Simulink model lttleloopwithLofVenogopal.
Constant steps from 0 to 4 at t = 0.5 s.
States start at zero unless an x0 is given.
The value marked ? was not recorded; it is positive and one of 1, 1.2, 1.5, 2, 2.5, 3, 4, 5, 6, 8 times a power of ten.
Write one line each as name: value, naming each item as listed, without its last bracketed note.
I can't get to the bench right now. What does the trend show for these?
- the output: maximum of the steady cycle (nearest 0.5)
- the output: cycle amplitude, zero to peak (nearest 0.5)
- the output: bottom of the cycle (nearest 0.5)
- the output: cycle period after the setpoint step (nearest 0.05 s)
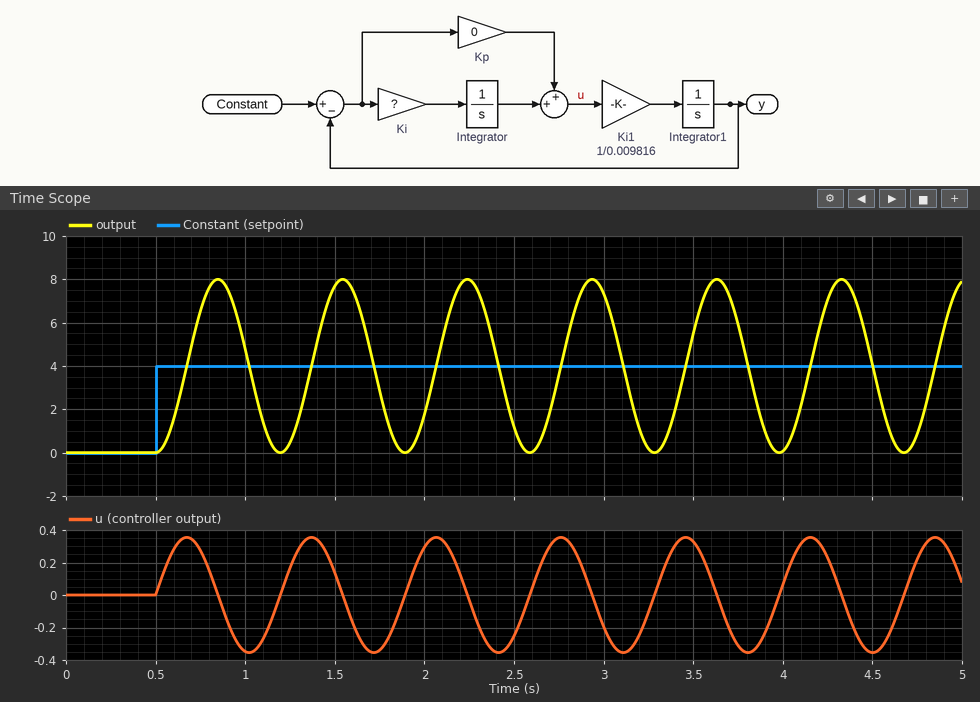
the output: maximum of the steady cycle: 8.0
the output: cycle amplitude, zero to peak: 4.0
the output: bottom of the cycle: 0.0
the output: cycle period after the setpoint step: 0.70 s
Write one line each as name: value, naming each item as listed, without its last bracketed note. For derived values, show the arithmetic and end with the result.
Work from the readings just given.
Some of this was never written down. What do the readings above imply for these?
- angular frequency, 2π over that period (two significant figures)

angular frequency, 2π over that period: 2π / 0.7 = 9.0 rad/s
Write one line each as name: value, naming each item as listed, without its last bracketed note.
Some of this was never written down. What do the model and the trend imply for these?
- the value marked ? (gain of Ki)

the value marked ?: 0.8
